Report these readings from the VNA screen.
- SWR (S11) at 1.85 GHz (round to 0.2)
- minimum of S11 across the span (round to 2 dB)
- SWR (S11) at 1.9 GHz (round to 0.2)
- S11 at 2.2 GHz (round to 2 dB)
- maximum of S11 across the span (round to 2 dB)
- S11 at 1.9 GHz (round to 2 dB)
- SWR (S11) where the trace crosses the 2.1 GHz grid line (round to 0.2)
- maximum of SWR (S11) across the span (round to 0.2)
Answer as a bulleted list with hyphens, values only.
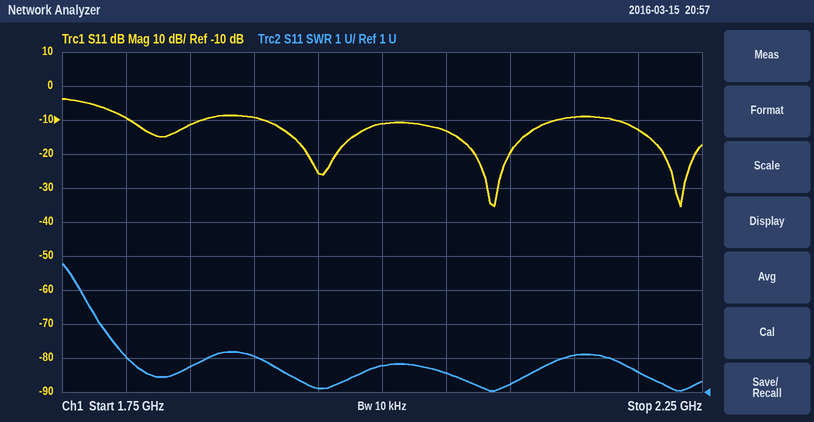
- 1.8
- -36 dB
- 2.0
- -12 dB
- -4 dB
- -10 dB
- 1.2
- 4.8
